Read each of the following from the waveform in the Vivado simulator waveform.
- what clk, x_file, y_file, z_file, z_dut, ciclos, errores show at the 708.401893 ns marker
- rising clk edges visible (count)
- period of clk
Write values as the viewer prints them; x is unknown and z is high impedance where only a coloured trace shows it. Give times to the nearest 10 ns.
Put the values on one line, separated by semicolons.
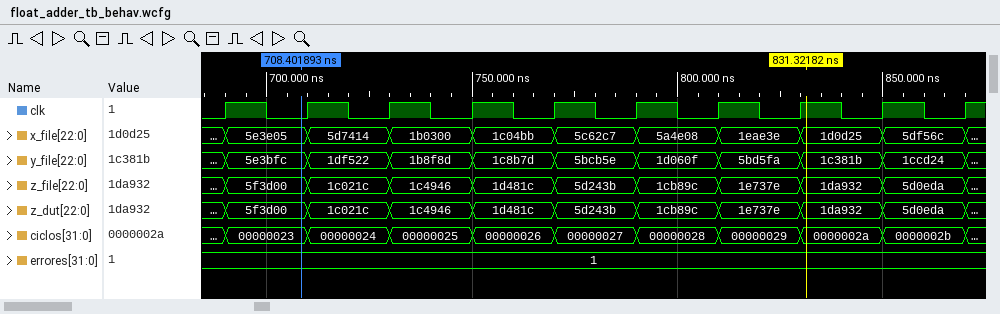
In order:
clk=0, x_file=5e3e05, y_file=5e3bfc, z_file=5f3d00, z_dut=5f3d00, ciclos=00000023, errores=1; 10; 20 ns
